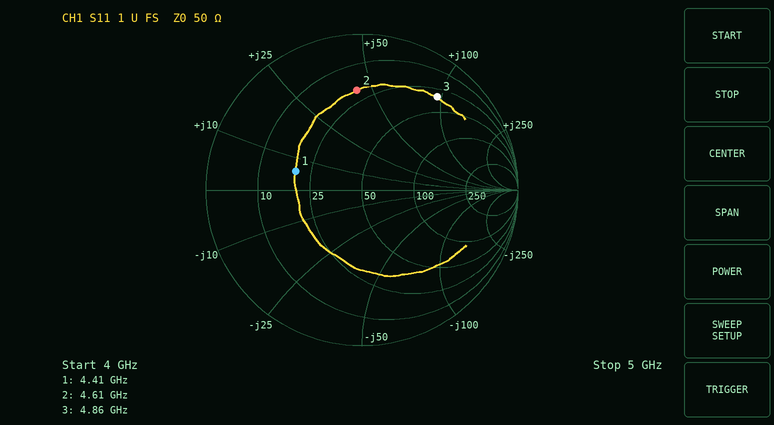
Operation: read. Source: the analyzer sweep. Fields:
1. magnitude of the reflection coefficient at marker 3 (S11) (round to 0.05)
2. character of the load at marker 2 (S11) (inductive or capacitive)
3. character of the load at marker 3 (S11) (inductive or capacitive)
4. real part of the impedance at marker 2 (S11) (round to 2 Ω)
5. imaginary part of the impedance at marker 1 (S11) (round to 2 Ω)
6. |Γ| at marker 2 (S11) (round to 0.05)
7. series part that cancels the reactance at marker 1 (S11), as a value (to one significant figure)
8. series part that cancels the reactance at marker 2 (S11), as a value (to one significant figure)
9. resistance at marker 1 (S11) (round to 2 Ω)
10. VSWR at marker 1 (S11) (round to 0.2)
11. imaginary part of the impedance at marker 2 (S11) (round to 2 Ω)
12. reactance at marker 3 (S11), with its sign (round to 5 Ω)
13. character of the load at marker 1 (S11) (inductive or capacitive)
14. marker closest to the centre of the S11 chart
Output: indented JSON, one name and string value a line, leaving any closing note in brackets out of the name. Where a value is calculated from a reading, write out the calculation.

{
  "magnitude of the reflection coefficient at marker 3 (S11)": "0.75",
  "character of the load at marker 2 (S11)": "inductive",
  "character of the load at marker 3 (S11)": "inductive",
  "real part of the impedance at marker 2 (S11)": "20 Ω",
  "imaginary part of the impedance at marker 1 (S11)": "+6 Ω",
  "|Γ| at marker 2 (S11)": "0.65",
  "series part that cancels the reactance at marker 1 (S11), as a value": "C = 1/(2π × 4.41 GHz × 6 Ω) ≈ 6 pF",
  "series part that cancels the reactance at marker 2 (S11), as a value": "C = 1/(2π × 4.61 GHz × 44 Ω) ≈ 785 fF, so 800 fF to one significant figure",
  "resistance at marker 1 (S11)": "20 Ω",
  "VSWR at marker 1 (S11)": "2.6",
  "imaginary part of the impedance at marker 2 (S11)": "+44 Ω",
  "reactance at marker 3 (S11), with its sign": "+95 Ω",
  "character of the load at marker 1 (S11)": "inductive",
  "marker closest to the centre of the S11 chart": "marker 1"
}
